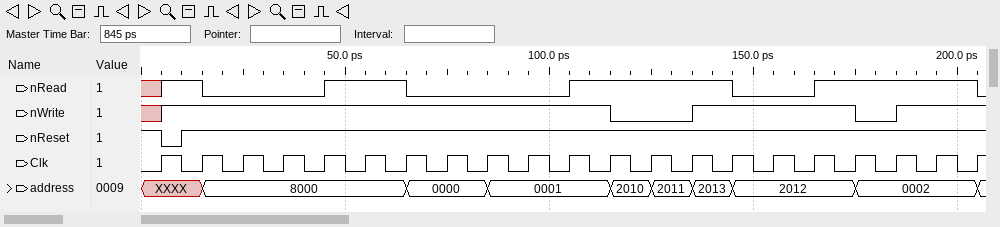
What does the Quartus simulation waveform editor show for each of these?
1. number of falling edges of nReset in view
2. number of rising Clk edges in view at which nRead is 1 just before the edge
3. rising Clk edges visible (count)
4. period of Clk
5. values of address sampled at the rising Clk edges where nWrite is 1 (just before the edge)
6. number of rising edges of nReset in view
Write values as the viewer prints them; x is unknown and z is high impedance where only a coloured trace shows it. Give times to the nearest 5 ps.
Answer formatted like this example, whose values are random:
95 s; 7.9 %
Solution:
1; 11; 21; 10 ps; XXXX, 8000, 8000, 8000, 8000, 8000, 0000, 0000, 0001, 0001, 0001, 2013, 2012, 2012, 2012, 0002, 0002; 1
